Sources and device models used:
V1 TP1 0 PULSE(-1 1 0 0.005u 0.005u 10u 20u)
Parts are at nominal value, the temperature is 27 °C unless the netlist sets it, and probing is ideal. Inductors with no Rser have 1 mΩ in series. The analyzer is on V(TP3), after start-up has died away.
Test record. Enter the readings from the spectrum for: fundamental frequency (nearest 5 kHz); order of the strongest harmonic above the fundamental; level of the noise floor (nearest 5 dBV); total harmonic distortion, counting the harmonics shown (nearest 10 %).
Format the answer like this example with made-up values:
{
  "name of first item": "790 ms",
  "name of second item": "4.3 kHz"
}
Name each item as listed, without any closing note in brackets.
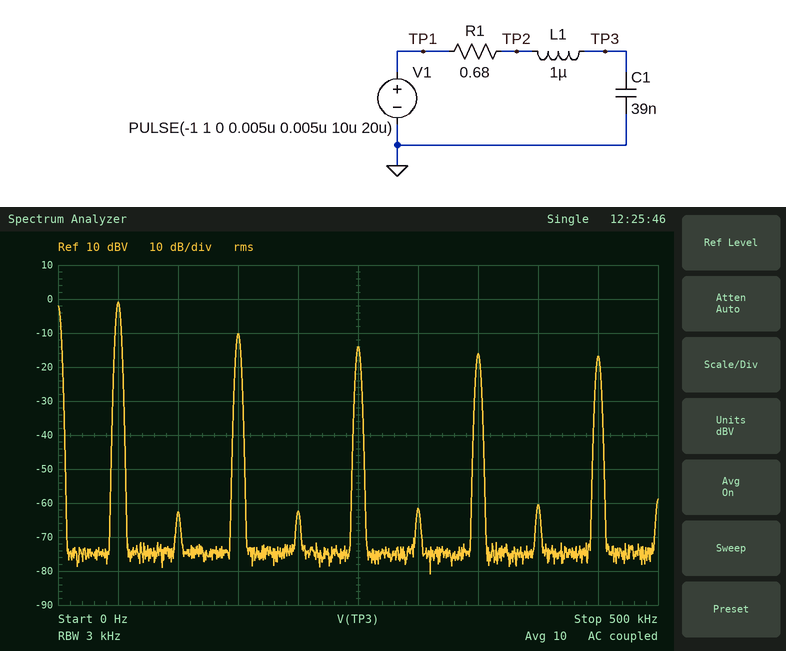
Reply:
{
  "fundamental frequency": "50 kHz",
  "order of the strongest harmonic above the fundamental": "3",
  "level of the noise floor": "-75 dBV",
  "total harmonic distortion, counting the harmonics shown": "50 %"
}
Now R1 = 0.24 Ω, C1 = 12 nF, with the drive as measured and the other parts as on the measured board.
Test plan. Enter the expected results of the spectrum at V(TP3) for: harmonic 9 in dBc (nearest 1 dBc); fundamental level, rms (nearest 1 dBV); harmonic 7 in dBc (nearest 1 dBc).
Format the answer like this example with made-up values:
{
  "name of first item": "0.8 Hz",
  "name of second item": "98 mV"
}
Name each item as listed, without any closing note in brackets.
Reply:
{
  "harmonic 9 in dBc": "-18 dBc",
  "fundamental level, rms": "-1 dBV",
  "harmonic 7 in dBc": "-16 dBc"
}
